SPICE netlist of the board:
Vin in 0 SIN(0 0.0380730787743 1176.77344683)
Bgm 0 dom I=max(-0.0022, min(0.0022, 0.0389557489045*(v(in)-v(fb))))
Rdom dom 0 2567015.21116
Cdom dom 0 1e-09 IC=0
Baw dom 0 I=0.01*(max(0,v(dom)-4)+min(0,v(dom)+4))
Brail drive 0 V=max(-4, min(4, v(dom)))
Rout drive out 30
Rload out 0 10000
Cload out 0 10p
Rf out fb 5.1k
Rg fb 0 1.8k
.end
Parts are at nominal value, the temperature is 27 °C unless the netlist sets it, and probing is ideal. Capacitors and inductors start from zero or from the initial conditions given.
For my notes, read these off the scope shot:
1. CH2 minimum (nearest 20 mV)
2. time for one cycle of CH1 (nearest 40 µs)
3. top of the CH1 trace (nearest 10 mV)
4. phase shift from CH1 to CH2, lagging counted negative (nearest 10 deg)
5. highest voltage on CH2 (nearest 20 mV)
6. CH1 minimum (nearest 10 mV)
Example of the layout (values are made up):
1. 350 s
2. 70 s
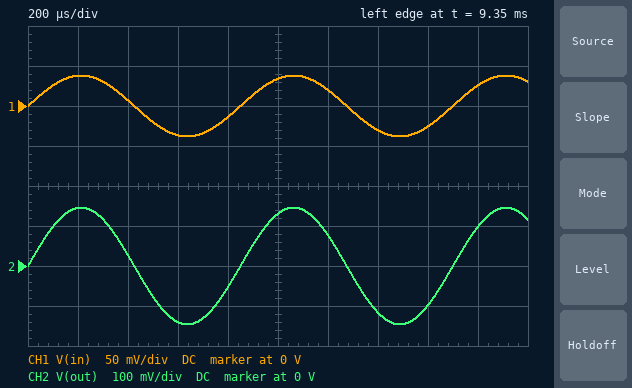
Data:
1. -140 mV
2. 840 µs
3. 40 mV
4. 0 deg
5. 140 mV
6. -40 mV
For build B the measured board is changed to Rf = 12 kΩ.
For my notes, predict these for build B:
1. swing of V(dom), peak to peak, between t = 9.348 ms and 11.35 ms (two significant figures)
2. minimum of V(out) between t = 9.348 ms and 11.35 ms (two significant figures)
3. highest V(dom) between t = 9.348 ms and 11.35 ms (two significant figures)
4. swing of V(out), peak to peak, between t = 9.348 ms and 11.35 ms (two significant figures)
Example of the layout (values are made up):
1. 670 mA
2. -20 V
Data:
1. 590 mV
2. -290 mV
3. 290 mV
4. 580 mV
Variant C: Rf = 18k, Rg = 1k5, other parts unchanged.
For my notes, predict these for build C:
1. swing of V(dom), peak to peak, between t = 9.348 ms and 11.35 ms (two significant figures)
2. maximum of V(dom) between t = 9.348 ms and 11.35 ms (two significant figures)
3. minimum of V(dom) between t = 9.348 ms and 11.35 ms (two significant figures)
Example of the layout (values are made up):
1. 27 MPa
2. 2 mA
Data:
1. 990 mV
2. 500 mV
3. -500 mV
